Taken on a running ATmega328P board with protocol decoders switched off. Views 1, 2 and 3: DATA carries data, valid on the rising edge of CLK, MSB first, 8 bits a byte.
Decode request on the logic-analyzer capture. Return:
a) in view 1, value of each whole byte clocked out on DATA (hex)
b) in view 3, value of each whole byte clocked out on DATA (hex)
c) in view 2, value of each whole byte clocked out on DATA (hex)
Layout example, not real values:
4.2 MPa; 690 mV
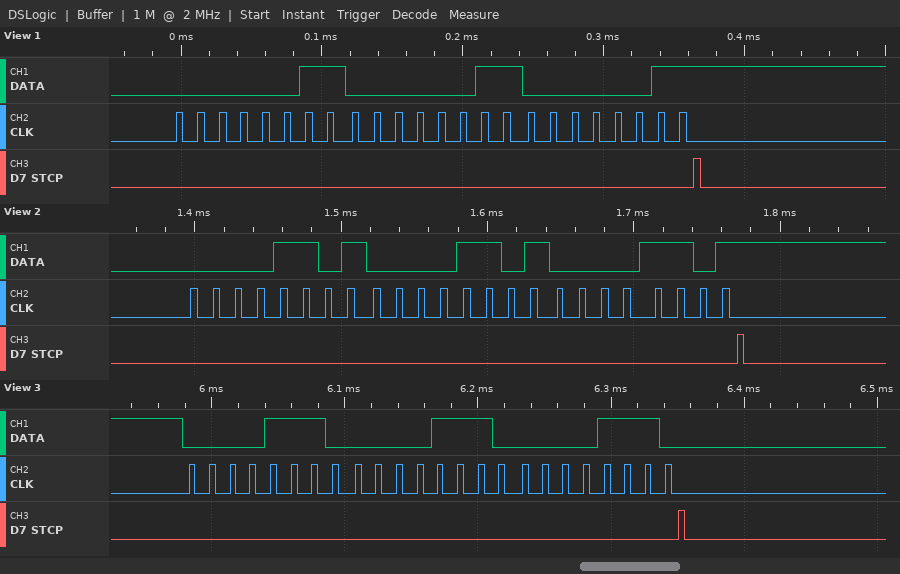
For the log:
03 03 03; 0E 0E 0E; 0D 0D 0D
